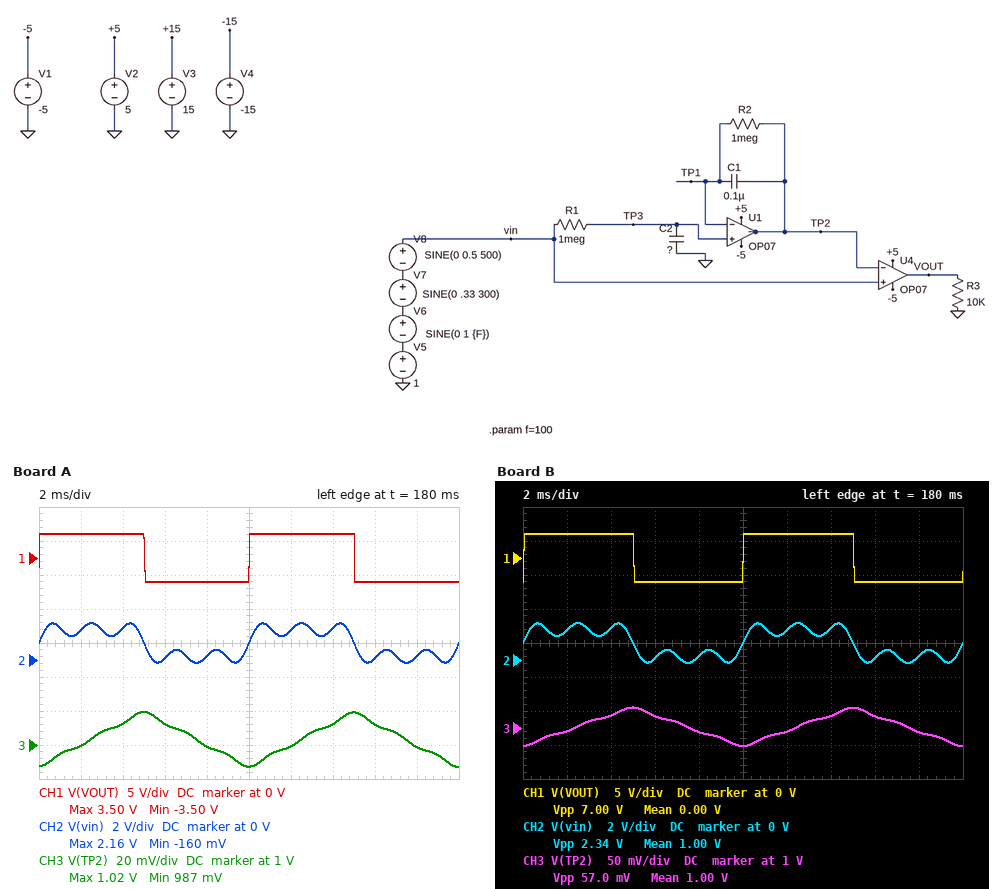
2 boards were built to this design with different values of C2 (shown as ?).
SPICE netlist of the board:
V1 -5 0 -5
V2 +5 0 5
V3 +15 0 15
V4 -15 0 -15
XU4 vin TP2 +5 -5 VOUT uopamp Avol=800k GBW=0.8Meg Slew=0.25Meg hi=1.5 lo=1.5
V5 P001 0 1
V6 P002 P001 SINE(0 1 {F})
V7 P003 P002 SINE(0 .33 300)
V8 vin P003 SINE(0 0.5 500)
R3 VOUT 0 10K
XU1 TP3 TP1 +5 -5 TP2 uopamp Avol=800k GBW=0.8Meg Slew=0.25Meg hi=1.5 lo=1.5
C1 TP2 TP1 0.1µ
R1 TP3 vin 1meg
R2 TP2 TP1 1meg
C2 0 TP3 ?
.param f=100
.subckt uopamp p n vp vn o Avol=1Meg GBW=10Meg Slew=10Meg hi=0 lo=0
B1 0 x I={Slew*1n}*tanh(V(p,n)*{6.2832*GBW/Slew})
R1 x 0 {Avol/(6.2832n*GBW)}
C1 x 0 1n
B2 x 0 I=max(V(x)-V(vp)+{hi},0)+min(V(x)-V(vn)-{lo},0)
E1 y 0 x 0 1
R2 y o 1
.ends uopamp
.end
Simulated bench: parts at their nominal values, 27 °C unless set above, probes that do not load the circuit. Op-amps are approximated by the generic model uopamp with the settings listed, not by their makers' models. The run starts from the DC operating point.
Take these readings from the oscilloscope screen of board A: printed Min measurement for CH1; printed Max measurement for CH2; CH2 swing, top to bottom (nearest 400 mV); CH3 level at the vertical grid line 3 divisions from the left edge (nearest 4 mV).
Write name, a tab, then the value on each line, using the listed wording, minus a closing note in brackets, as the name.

printed Min measurement for CH1	-3.50 V
printed Max measurement for CH2	2.16 V
CH2 swing, top to bottom	2.4 V
CH3 level at the vertical grid line 3 divisions from the left edge	1.012 V
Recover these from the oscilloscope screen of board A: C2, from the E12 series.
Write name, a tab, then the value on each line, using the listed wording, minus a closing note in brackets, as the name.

C2, from the E12 series	120 nF
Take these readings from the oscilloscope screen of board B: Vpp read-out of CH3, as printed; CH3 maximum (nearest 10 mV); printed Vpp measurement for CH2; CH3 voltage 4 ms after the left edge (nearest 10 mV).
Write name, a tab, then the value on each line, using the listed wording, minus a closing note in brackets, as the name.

Vpp read-out of CH3, as printed	57.0 mV
CH3 maximum	1.03 V
printed Vpp measurement for CH2	2.34 V
CH3 voltage 4 ms after the left edge	1.02 V
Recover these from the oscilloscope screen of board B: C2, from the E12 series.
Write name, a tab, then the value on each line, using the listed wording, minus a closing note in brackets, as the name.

C2, from the E12 series	68 nF
